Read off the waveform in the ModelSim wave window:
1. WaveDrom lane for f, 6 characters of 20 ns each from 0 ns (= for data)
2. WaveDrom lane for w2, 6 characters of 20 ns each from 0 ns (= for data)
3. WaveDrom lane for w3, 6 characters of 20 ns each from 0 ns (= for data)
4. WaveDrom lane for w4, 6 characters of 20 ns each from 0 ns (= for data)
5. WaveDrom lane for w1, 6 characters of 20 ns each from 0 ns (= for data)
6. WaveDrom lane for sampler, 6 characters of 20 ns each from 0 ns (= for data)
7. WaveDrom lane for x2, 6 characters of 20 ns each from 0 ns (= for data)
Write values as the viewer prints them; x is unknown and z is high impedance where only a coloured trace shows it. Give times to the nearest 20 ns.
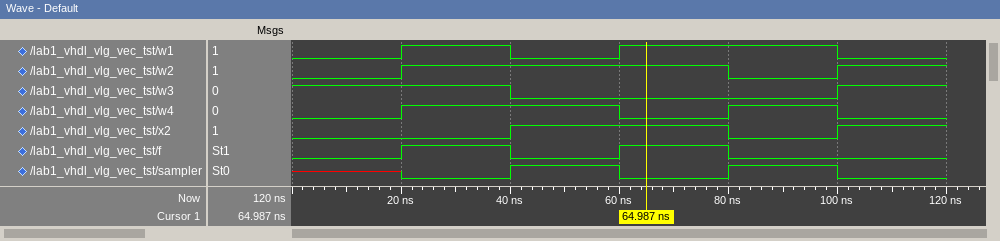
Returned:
{name: 'f', wave: '01010.'}
{name: 'w2', wave: '01..01'}
{name: 'w3', wave: '1.0..1'}
{name: 'w4', wave: '01.010'}
{name: 'w1', wave: '0101.0'}
{name: 'sampler', wave: 'x01010'}
{name: 'x2', wave: '0.1.01'}
